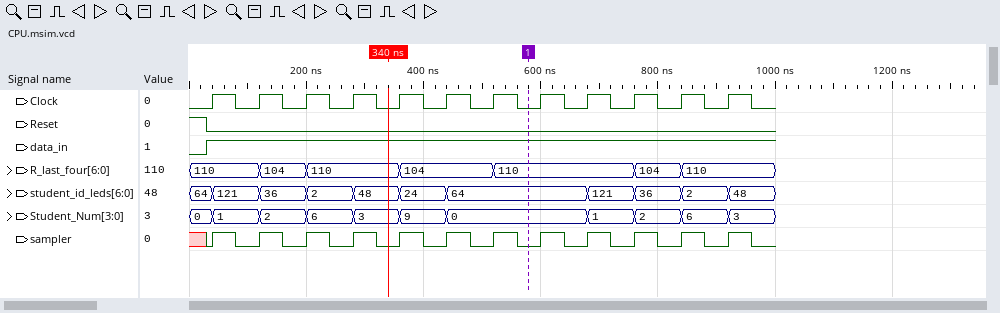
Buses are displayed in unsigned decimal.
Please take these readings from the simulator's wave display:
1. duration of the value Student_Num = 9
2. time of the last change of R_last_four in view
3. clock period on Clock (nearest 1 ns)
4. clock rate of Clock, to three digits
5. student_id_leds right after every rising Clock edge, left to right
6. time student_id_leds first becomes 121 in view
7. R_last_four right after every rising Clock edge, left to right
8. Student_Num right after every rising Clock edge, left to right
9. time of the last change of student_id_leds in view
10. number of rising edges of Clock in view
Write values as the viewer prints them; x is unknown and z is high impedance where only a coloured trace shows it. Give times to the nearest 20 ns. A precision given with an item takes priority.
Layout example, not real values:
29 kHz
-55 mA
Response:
80 ns
840 ns
80 ns
12.5 MHz
121, 36, 2, 48, 24, 64, 64, 64, 121, 36, 2, 48
40 ns
110, 104, 110, 110, 104, 104, 110, 110, 110, 104, 110, 110
1, 2, 6, 3, 9, 0, 0, 0, 1, 2, 6, 3
920 ns
12
